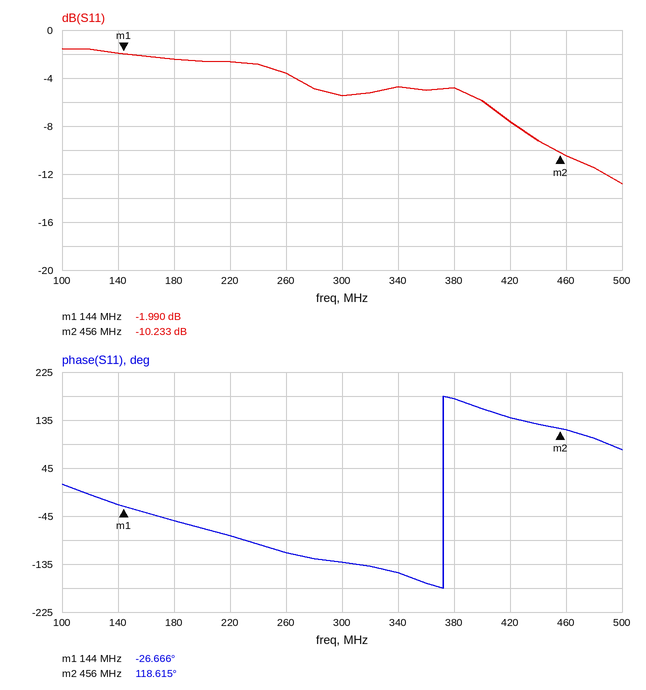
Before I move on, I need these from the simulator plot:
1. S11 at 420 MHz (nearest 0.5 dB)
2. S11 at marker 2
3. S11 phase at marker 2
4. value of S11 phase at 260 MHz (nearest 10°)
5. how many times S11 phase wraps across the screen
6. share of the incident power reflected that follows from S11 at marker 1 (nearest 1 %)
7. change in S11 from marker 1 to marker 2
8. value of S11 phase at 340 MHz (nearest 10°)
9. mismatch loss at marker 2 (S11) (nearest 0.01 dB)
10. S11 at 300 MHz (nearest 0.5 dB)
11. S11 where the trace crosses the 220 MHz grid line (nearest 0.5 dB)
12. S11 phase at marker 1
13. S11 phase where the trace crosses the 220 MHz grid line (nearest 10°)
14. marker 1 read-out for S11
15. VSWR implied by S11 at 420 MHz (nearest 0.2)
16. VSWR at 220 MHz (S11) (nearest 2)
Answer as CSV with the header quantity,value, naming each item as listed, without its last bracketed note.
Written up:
quantity,value
S11 at 420 MHz,-7.5 dB
S11 at marker 2,-10.233 dB
S11 phase at marker 2,118.615°
value of S11 phase at 260 MHz,-110°
how many times S11 phase wraps across the screen,1
share of the incident power reflected that follows from S11 at marker 1,63 %
change in S11 from marker 1 to marker 2,-8.243 dB
value of S11 phase at 340 MHz,-150°
mismatch loss at marker 2 (S11),0.43 dB
S11 at 300 MHz,-5.5 dB
S11 where the trace crosses the 220 MHz grid line,-2.5 dB
S11 phase at marker 1,-26.666°
S11 phase where the trace crosses the 220 MHz grid line,-80°
marker 1 read-out for S11,-1.990 dB
VSWR implied by S11 at 420 MHz,2.4
VSWR at 220 MHz (S11),6
